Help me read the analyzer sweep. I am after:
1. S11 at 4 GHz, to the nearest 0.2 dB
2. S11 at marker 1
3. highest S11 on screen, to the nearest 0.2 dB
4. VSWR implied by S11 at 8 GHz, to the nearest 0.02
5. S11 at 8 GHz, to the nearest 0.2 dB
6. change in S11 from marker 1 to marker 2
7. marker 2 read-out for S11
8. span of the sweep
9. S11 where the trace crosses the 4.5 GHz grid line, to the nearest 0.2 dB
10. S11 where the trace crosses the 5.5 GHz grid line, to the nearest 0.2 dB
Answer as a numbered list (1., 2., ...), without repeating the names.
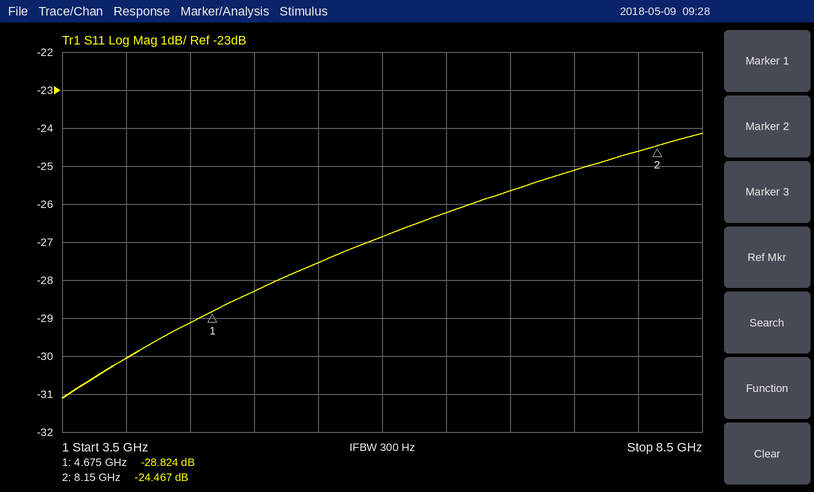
1. -30.0 dB
2. -28.824 dB
3. -24.2 dB
4. 1.12
5. -24.6 dB
6. 4.357 dB
7. -24.467 dB
8. 5 GHz
9. -29.2 dB
10. -27.6 dB
